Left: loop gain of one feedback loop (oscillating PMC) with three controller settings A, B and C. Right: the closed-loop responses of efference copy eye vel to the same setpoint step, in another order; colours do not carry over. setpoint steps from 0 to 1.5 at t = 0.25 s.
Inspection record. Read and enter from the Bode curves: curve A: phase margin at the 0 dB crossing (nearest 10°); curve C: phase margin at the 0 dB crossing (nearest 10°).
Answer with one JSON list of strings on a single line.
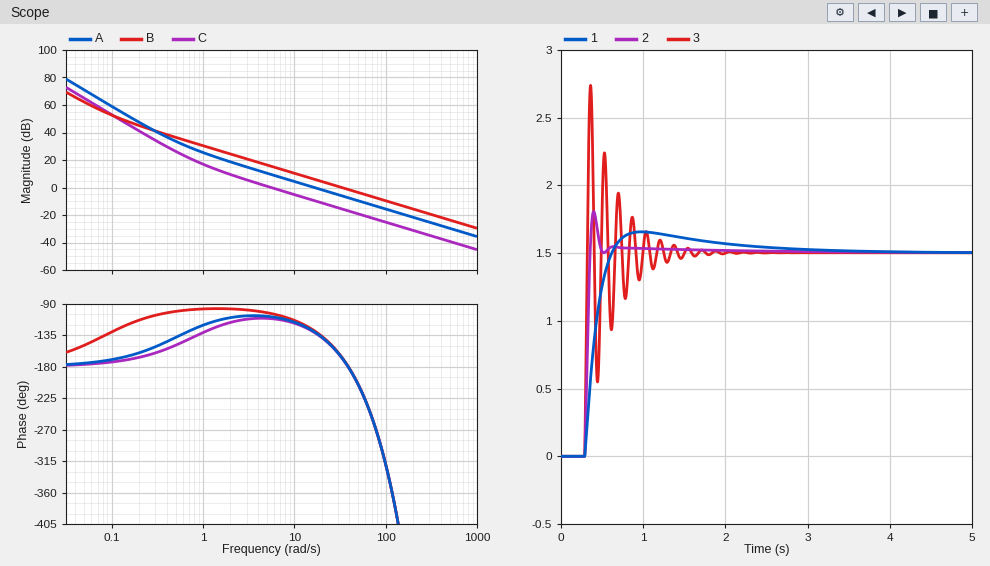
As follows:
["50°", "70°"]
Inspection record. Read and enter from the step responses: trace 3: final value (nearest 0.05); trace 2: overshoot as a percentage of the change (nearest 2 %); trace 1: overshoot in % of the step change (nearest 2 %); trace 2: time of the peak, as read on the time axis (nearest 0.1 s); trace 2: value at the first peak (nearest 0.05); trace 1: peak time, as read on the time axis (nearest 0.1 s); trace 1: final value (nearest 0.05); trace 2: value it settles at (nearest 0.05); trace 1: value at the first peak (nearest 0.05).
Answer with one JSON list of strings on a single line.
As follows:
["1.50", "20 %", "10 %", "0.4 s", "1.80", "1.0 s", "1.50", "1.50", "1.65"]
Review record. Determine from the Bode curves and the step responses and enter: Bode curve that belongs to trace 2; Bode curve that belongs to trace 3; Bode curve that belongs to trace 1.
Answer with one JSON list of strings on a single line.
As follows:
["A", "B", "C"]
